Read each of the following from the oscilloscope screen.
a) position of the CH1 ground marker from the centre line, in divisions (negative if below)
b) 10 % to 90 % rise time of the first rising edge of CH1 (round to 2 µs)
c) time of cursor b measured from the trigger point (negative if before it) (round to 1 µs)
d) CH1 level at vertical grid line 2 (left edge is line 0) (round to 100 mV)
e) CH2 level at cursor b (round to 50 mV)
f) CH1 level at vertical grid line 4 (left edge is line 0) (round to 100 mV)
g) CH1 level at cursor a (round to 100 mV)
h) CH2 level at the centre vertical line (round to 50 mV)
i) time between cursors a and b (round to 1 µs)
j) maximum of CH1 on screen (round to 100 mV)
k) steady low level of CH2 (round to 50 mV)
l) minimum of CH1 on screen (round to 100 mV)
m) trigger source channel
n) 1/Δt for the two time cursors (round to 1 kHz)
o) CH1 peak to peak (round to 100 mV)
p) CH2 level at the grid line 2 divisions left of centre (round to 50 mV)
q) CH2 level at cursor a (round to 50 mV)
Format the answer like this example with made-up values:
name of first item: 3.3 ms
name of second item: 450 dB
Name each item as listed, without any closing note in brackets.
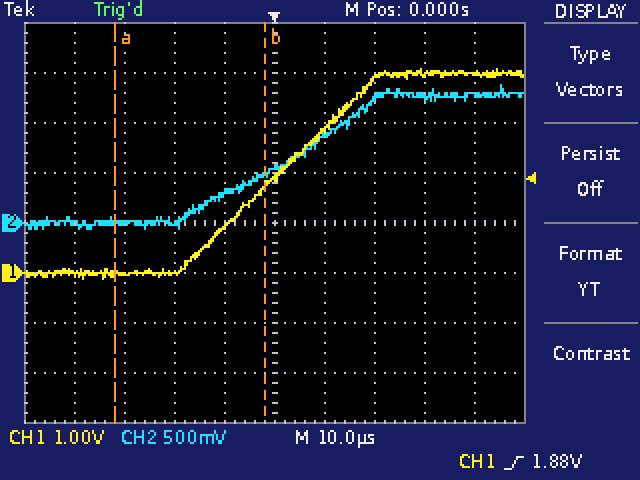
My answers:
position of the CH1 ground marker from the centre line, in divisions: -1.0 div
10 % to 90 % rise time of the first rising edge of CH1: 32 µs
time of cursor b measured from the trigger point (negative if before it): -2 µs
CH1 level at vertical grid line 2 (left edge is line 0): 0.0 V
CH2 level at cursor b: 500 mV
CH1 level at vertical grid line 4 (left edge is line 0): 900 mV
CH1 level at cursor a: 0.0 V
CH2 level at the centre vertical line: 550 mV
time between cursors a and b: 30 µs
maximum of CH1 on screen: 4.1 V
steady low level of CH2: 0 mV
minimum of CH1 on screen: -100 mV
trigger source channel: CH1
1/Δt for the two time cursors: 33 kHz
CH1 peak to peak: 4.2 V
CH2 level at the grid line 2 divisions left of centre: 0 mV
CH2 level at cursor a: 0 mV
